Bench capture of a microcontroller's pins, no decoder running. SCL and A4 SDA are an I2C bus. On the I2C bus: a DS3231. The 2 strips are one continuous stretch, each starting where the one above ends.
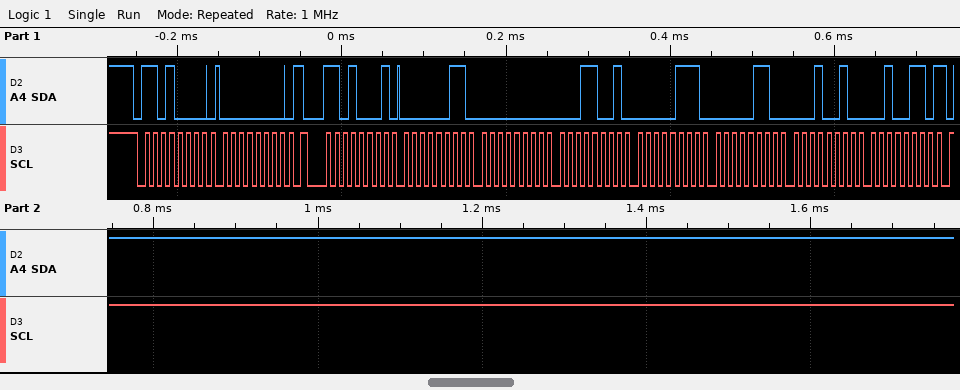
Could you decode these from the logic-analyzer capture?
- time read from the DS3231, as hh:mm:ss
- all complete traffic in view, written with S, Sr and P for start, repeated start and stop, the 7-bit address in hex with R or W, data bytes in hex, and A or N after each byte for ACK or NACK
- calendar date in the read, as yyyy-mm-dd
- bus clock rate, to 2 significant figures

19:00:03
S 68W A 00 A Sr 68R A 03 A 00 A 19 A 07 A 06 A 12 A 26 N P
2026-12-06
100 kHz
